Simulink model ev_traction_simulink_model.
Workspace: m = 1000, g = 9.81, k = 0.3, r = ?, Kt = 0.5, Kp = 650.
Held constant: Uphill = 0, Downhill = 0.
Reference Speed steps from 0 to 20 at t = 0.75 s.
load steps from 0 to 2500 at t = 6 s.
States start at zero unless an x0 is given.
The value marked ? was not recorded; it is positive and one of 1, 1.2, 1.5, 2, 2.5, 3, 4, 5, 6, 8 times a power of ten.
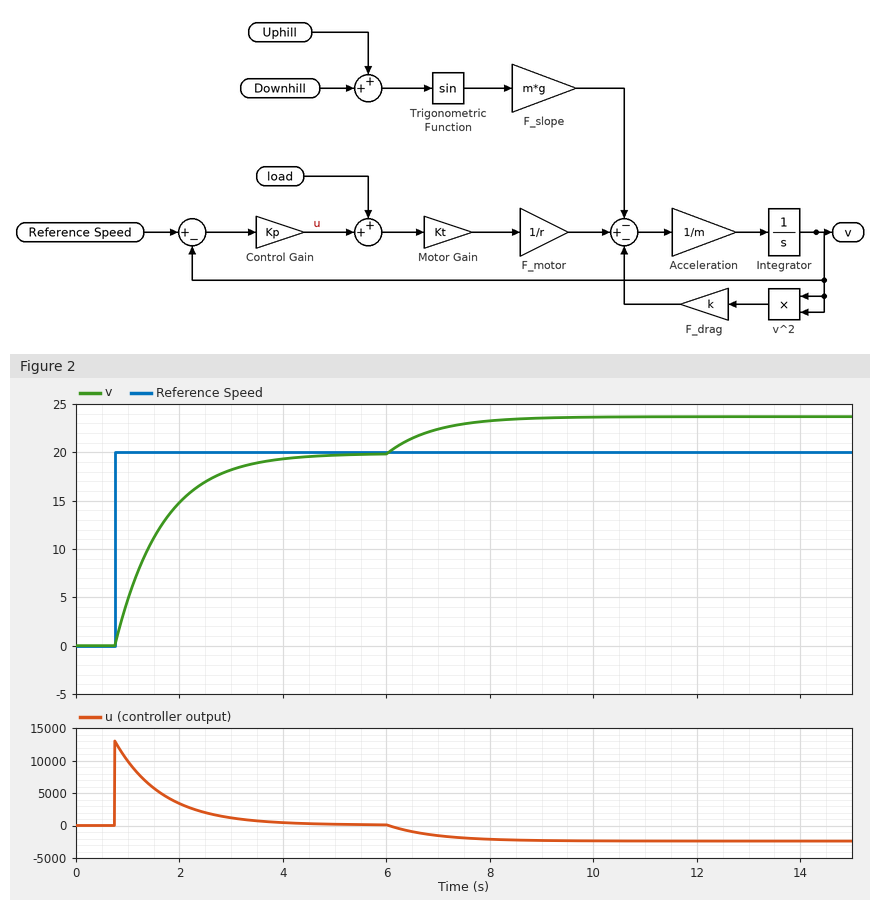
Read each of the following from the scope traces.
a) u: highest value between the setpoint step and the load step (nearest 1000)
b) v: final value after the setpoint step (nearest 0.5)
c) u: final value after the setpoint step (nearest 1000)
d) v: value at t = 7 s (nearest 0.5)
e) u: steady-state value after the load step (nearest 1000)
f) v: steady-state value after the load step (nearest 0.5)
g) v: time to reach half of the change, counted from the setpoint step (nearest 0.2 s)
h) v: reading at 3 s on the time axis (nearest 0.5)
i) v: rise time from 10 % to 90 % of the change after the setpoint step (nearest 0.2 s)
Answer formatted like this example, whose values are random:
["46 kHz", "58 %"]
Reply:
["13000", "20.0", "0", "22.5", "-2000", "23.5", "0.6 s", "18.0", "2.0 s"]
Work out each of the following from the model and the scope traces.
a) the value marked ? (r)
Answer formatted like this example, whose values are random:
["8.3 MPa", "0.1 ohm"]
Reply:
["0.3"]
